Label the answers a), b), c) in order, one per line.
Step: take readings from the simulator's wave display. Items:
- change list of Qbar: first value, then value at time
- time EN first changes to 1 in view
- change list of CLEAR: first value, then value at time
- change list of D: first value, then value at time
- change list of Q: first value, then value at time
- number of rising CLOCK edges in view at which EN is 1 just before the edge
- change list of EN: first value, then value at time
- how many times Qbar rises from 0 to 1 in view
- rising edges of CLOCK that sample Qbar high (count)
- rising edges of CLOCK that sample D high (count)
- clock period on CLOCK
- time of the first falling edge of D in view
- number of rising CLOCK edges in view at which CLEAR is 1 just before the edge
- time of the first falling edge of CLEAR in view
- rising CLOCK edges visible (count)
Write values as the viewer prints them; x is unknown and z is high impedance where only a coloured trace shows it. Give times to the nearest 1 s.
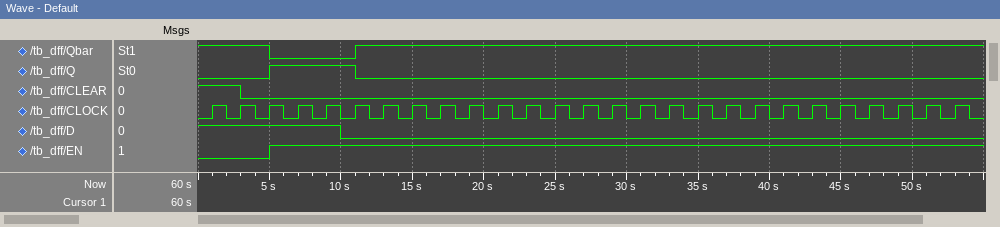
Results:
a) 1, 0 at 5 s, 1 at 11 s
b) 5 s
c) 1, 0 at 3 s
d) 1, 0 at 10 s
e) 0, 1 at 5 s, 0 at 11 s
f) 24
g) 0, 1 at 5 s
h) 1
i) 24
j) 5
k) 2 s
l) 10 s
m) 2
n) 3 s
o) 27
